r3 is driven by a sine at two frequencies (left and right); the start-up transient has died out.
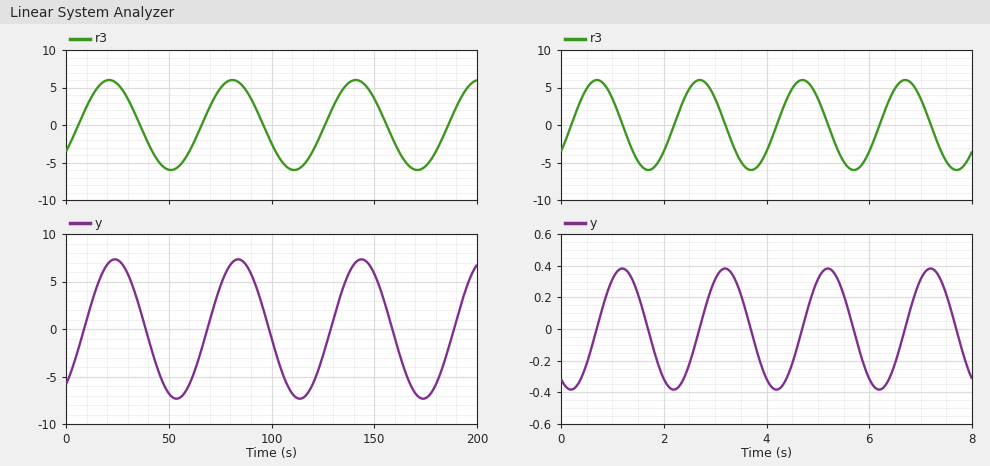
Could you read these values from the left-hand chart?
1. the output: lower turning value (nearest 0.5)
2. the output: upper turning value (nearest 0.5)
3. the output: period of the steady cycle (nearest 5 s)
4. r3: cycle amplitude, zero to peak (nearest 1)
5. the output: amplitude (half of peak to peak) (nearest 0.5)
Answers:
-7.5
7.5
60 s
6
7.5
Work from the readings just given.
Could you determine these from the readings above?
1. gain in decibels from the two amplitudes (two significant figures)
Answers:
1.9 dB
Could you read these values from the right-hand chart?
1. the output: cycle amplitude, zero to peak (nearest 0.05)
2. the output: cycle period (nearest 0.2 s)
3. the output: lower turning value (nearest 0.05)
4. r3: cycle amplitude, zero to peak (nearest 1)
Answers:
0.40
2.0 s
-0.40
6
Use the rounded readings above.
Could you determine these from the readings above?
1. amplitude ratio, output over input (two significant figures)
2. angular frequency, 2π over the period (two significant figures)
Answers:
0.067
3.1 rad/s
